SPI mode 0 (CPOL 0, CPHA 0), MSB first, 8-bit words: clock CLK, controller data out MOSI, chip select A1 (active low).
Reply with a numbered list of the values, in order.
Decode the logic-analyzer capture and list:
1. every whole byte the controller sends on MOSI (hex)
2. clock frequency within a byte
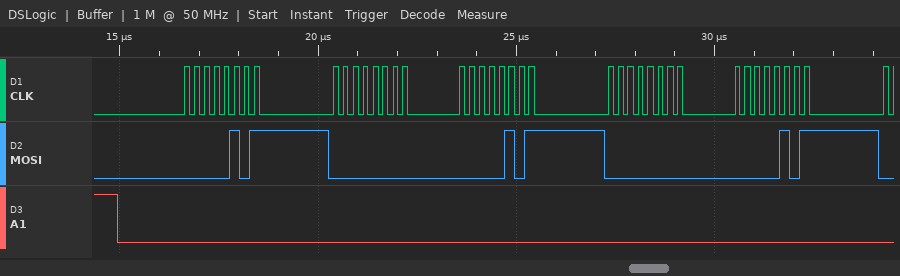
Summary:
1. 0x05 0x00 0x05 0x00 0x05
2. 4 MHz
